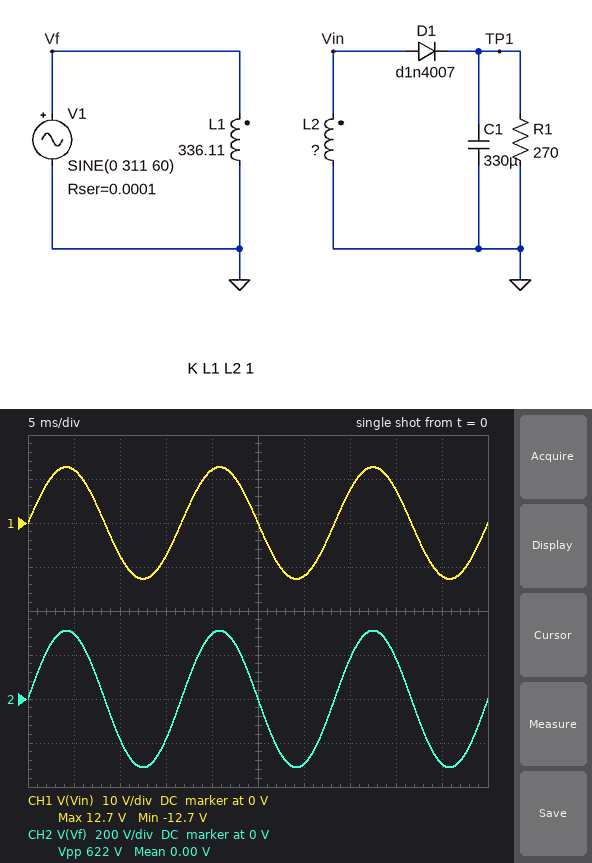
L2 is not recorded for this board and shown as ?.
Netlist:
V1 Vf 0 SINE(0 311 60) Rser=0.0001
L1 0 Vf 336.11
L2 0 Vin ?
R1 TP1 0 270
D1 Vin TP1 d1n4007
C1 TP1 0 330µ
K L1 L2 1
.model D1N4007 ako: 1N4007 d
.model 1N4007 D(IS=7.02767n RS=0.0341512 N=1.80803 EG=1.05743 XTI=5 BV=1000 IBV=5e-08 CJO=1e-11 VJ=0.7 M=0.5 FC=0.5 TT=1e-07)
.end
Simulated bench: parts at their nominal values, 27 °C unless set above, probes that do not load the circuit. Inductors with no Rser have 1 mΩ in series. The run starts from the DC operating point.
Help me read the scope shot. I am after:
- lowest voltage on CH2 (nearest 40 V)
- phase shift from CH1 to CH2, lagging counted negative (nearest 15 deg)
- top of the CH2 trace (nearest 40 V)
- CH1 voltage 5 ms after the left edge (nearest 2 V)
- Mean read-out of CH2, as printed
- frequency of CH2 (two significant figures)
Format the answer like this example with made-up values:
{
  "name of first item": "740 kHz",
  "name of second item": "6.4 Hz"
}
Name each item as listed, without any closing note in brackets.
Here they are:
{
  "lowest voltage on CH2": "-320 V",
  "phase shift from CH1 to CH2, lagging counted negative": "0 deg",
  "top of the CH2 trace": "320 V",
  "CH1 voltage 5 ms after the left edge": "12 V",
  "Mean read-out of CH2, as printed": "0.00 V",
  "frequency of CH2": "60 Hz"
}
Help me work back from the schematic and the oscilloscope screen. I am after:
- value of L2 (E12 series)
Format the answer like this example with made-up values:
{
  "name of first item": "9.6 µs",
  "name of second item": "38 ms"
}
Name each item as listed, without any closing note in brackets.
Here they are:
{
  "value of L2": "560 mH"
}
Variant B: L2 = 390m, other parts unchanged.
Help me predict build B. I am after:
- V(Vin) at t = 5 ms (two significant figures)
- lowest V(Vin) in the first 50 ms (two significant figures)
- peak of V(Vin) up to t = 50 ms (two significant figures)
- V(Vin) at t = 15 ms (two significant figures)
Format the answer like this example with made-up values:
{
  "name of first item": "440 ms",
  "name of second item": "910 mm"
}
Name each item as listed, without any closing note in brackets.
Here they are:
{
  "V(Vin) at t = 5 ms": "10 V",
  "lowest V(Vin) in the first 50 ms": "-11 V",
  "peak of V(Vin) up to t = 50 ms": "11 V",
  "V(Vin) at t = 15 ms": "-6.2 V"
}
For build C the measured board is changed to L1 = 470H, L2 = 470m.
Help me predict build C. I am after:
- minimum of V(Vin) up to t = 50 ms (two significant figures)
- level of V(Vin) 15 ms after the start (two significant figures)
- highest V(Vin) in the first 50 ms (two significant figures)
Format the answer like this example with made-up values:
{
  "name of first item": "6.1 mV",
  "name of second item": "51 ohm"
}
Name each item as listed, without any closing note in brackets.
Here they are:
{
  "minimum of V(Vin) up to t = 50 ms": "-9.8 V",
  "level of V(Vin) 15 ms after the start": "-5.8 V",
  "highest V(Vin) in the first 50 ms": "9.8 V"
}
